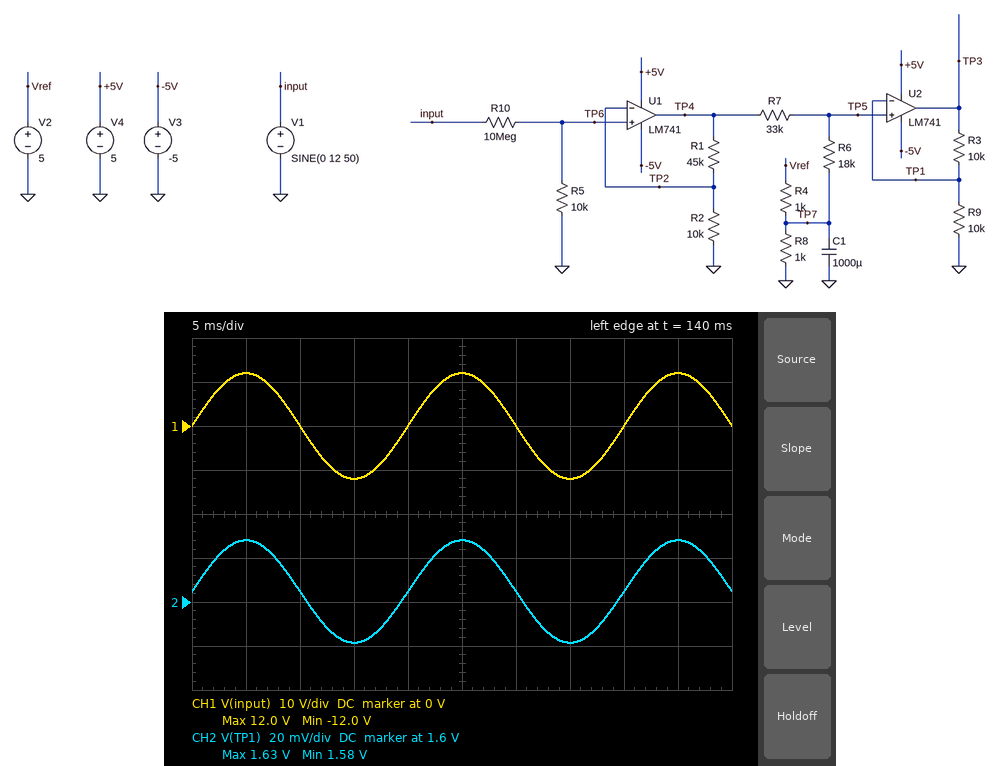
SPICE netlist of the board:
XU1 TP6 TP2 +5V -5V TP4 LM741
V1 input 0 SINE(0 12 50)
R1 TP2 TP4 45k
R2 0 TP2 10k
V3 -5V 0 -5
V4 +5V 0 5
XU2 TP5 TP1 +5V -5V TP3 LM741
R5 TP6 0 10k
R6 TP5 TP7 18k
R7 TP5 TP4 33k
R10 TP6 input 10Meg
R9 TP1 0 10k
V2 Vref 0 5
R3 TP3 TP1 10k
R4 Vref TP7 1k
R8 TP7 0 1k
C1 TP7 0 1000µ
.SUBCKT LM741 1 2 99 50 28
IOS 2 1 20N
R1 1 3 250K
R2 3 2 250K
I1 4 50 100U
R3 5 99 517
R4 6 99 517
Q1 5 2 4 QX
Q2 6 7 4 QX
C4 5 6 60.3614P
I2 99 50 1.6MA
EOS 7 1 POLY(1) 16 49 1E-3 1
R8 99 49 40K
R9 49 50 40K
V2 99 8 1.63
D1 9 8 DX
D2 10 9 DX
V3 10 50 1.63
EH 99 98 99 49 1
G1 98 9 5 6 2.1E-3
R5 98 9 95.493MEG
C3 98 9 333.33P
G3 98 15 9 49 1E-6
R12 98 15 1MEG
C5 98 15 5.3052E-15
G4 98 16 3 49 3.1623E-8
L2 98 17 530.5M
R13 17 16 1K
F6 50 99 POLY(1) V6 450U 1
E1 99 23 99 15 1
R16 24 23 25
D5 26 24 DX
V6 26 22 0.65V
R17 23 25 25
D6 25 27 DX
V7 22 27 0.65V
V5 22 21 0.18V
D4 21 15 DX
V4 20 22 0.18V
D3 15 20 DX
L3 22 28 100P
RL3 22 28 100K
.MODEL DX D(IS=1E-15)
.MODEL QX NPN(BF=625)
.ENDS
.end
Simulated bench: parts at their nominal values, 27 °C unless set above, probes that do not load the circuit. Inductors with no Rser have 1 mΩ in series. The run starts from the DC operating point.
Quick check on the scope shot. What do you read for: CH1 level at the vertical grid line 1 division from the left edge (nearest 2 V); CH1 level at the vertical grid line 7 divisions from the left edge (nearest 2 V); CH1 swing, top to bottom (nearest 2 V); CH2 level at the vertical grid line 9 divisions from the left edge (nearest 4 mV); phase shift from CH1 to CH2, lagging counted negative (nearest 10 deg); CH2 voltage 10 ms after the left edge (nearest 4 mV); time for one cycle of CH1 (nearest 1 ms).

12 V
-12 V
24 V
1.628 V
0 deg
1.604 V
20 ms
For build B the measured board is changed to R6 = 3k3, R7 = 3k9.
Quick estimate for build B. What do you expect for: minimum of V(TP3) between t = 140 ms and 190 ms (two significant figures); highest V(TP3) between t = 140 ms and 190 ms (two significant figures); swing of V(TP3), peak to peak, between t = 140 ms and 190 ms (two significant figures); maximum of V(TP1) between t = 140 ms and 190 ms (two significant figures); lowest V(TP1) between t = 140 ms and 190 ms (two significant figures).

2.5 V
2.6 V
120 mV
1.3 V
1.2 V
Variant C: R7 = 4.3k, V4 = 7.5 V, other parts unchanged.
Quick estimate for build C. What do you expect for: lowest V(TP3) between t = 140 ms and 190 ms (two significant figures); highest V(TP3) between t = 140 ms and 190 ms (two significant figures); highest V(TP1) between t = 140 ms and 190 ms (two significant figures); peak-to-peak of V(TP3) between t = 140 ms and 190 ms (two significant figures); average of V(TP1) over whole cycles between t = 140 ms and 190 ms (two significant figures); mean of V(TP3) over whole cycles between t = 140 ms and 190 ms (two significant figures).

850 mV
1.1 V
530 mV
210 mV
480 mV
960 mV
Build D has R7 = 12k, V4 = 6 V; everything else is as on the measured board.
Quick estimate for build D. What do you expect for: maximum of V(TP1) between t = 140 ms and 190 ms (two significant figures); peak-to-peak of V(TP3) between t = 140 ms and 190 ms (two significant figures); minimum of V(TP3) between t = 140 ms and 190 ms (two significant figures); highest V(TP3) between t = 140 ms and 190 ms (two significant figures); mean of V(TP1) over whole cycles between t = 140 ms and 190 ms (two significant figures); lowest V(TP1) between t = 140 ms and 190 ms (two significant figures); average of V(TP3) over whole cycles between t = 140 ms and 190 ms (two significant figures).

1.0 V
160 mV
1.9 V
2.1 V
990 mV
950 mV
2.0 V
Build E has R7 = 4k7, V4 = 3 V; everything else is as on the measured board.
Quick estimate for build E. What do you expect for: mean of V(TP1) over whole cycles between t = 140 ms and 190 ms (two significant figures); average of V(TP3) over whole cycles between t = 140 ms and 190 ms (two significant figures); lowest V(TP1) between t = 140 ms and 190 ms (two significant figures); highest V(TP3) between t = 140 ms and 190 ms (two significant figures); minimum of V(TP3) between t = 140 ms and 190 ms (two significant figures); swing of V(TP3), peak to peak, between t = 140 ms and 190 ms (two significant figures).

510 mV
1.0 V
460 mV
1.1 V
920 mV
210 mV
